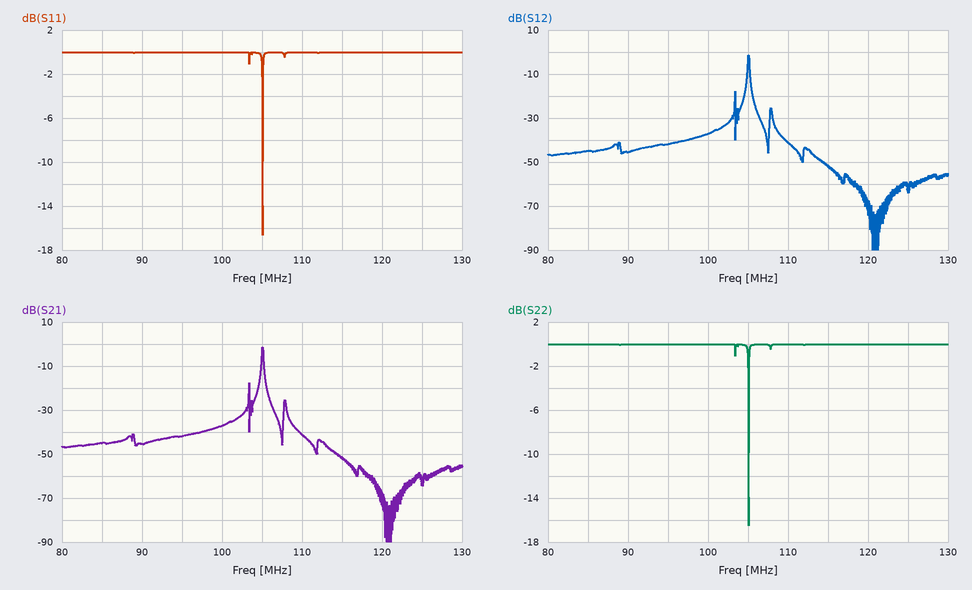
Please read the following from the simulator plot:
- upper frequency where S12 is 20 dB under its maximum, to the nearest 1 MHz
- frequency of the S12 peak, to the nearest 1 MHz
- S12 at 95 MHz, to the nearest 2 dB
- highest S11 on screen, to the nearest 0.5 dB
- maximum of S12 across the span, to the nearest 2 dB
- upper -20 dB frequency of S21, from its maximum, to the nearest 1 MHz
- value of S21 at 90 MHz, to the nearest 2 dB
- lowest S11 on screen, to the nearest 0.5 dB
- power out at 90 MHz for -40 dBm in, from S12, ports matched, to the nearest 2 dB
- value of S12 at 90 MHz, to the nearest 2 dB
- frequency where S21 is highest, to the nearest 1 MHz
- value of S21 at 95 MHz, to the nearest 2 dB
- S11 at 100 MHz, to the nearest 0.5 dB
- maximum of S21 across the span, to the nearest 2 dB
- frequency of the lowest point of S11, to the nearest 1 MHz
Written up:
106 MHz
105 MHz
-42 dB
0.0 dB
-2 dB
106 MHz
-46 dB
-16.5 dB
-86 dBm
-46 dB
105 MHz
-42 dB
0.0 dB
-2 dB
105 MHz
